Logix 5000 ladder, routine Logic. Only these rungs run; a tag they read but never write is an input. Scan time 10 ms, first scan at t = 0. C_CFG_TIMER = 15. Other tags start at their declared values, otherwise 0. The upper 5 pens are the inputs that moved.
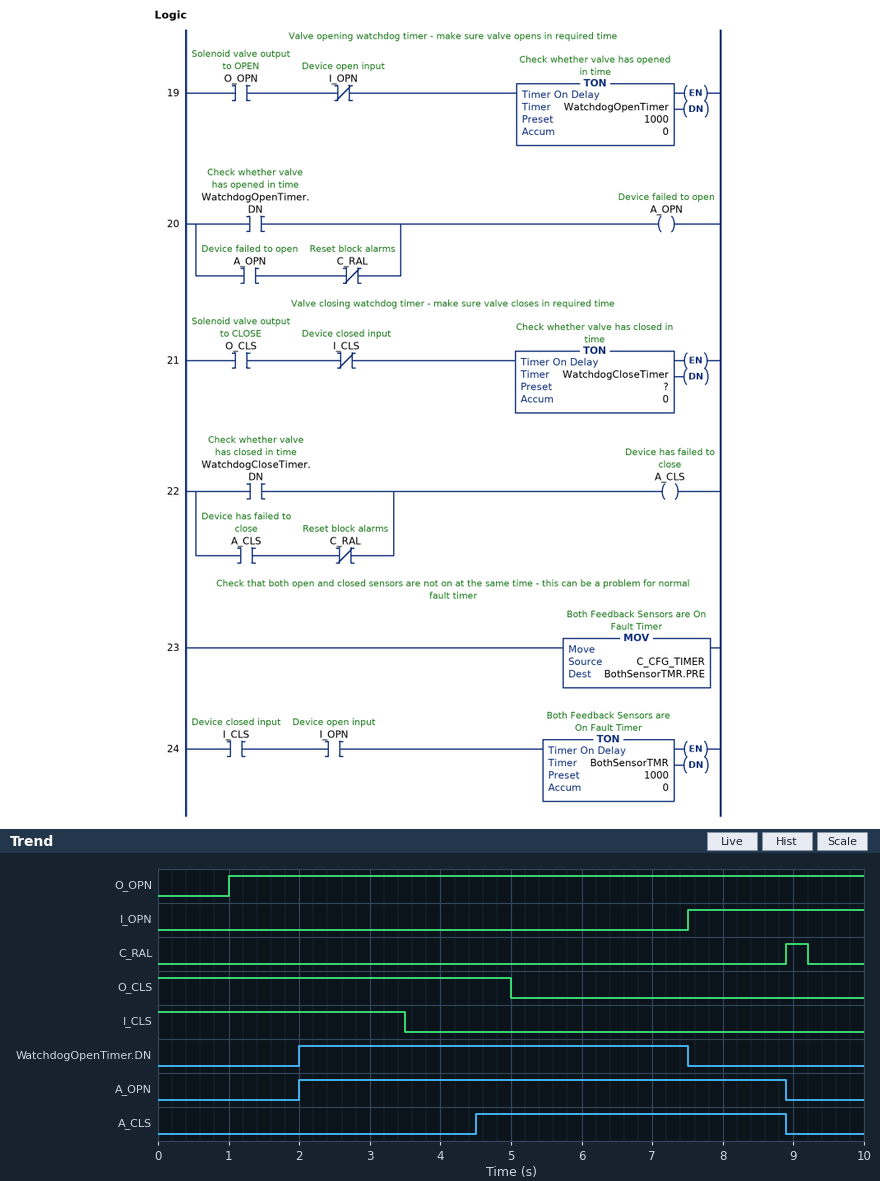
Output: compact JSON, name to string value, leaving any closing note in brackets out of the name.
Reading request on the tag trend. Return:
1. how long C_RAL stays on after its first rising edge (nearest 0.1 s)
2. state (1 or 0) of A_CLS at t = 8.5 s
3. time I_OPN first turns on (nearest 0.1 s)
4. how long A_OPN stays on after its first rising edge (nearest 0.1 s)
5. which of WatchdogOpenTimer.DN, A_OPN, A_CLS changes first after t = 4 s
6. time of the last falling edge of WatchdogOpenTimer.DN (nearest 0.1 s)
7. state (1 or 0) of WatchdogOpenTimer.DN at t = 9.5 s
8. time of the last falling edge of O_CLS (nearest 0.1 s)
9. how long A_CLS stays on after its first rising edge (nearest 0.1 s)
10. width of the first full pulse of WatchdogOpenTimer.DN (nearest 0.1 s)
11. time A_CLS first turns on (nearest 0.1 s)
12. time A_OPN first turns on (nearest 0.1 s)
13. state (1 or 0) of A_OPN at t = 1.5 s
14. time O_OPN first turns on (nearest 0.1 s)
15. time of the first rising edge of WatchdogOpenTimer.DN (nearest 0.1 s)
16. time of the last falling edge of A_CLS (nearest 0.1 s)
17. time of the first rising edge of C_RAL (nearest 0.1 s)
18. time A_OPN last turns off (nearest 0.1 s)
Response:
{"how long C_RAL stays on after its first rising edge": "0.3 s", "state (1 or 0) of A_CLS at t = 8.5 s": "1", "time I_OPN first turns on": "7.5 s", "how long A_OPN stays on after its first rising edge": "6.9 s", "which of WatchdogOpenTimer.DN, A_OPN, A_CLS changes first after t = 4 s": "A_CLS", "time of the last falling edge of WatchdogOpenTimer.DN": "7.5 s", "state (1 or 0) of WatchdogOpenTimer.DN at t = 9.5 s": "0", "time of the last falling edge of O_CLS": "5.0 s", "how long A_CLS stays on after its first rising edge": "4.4 s", "width of the first full pulse of WatchdogOpenTimer.DN": "5.5 s", "time A_CLS first turns on": "4.5 s", "time A_OPN first turns on": "2.0 s", "state (1 or 0) of A_OPN at t = 1.5 s": "0", "time O_OPN first turns on": "1.0 s", "time of the first rising edge of WatchdogOpenTimer.DN": "2.0 s", "time of the last falling edge of A_CLS": "8.9 s", "time of the first rising edge of C_RAL": "8.9 s", "time A_OPN last turns off": "8.9 s"}
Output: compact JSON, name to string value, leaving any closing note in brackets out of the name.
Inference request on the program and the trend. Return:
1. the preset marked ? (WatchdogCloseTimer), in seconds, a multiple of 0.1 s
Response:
{"the preset marked ? (WatchdogCloseTimer), in seconds, a multiple of 0.1 s": "1.0 s"}
